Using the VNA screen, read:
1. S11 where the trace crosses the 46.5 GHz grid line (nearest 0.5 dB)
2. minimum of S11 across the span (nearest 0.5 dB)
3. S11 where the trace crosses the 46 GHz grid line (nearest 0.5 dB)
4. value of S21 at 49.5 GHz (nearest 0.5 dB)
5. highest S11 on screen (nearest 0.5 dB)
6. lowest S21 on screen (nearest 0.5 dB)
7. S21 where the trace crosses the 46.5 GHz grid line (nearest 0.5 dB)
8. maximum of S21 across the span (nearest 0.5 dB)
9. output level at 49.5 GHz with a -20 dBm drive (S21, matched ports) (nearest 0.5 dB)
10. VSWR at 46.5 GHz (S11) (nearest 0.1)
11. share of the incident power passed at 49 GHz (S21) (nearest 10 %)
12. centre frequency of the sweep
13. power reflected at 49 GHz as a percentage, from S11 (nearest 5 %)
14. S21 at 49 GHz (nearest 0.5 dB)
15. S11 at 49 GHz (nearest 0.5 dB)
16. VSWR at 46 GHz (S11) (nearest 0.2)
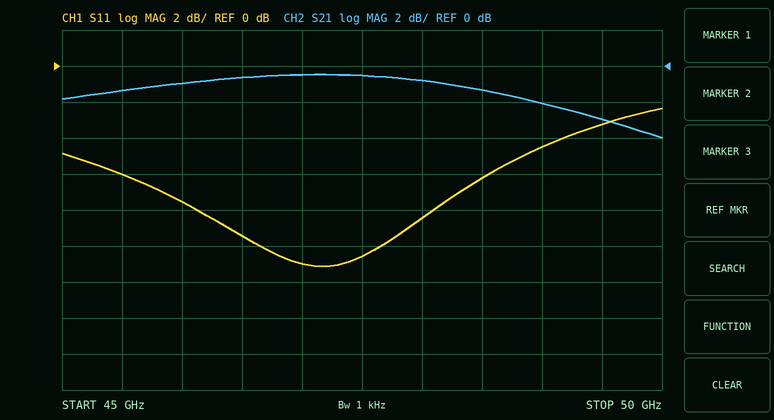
-9.5 dB
-11.0 dB
-7.5 dB
-3.0 dB
-2.5 dB
-4.0 dB
-0.5 dB
-0.5 dB
-23.0 dBm
2.0
60 %
47.5 GHz
35 %
-2.0 dB
-4.5 dB
2.4
